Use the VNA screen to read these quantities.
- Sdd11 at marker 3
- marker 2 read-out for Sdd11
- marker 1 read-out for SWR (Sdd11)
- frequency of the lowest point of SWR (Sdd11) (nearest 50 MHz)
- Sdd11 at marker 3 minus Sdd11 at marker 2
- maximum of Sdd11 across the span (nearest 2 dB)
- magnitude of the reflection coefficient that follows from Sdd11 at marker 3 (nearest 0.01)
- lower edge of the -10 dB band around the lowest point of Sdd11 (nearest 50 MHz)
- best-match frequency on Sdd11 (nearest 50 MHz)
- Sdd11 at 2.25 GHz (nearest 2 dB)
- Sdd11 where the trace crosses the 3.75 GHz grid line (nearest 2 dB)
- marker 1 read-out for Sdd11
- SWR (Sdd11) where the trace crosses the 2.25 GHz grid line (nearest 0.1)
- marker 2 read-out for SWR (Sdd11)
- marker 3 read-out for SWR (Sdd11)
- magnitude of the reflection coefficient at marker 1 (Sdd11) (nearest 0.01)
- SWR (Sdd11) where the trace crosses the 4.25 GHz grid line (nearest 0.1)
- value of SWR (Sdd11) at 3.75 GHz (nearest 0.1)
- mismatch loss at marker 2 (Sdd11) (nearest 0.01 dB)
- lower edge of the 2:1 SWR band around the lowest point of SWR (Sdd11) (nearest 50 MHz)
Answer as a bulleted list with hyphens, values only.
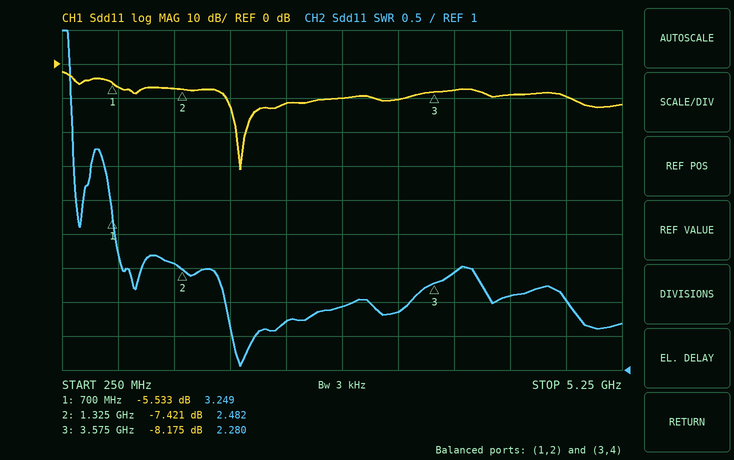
- -8.175 dB
- -7.421 dB
- 3.249
- 1.85 GHz
- -0.754 dB
- -2 dB
- 0.39
- 1.70 GHz
- 1.85 GHz
- -12 dB
- -8 dB
- -5.533 dB
- 1.7
- 2.482
- 2.280
- 0.53
- 2.1
- 2.4
- 0.87 dB
- 1.70 GHz
